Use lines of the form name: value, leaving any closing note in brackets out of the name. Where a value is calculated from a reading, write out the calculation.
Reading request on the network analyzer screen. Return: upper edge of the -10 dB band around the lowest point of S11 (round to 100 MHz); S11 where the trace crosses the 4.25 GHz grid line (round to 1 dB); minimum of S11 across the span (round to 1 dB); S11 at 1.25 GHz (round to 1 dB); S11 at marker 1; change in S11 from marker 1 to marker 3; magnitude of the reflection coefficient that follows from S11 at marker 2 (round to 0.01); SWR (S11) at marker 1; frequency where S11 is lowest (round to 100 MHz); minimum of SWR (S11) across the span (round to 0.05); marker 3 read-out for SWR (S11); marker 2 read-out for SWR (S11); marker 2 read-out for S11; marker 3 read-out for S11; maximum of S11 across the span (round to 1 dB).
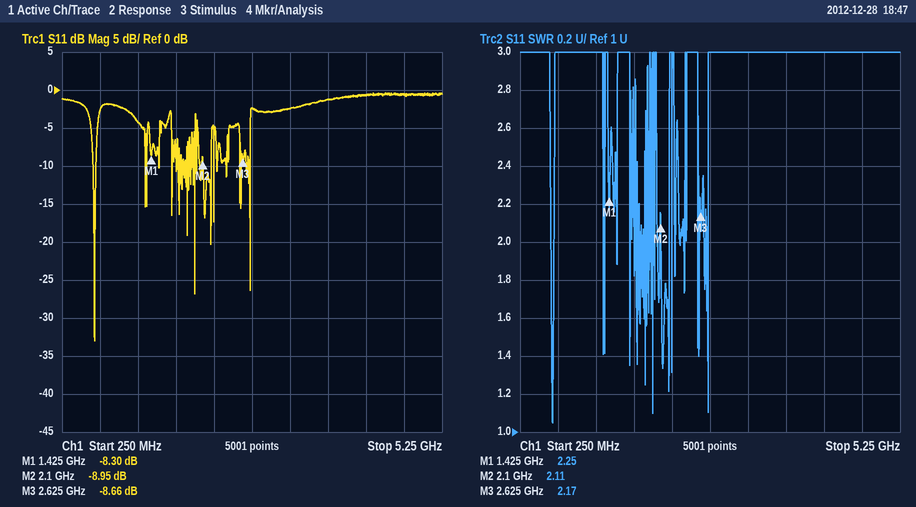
upper edge of the -10 dB band around the lowest point of S11: 700 MHz
S11 where the trace crosses the 4.25 GHz grid line: -1 dB
minimum of S11 across the span: -33 dB
S11 at 1.25 GHz: -4 dB
S11 at marker 1: -8.30 dB
change in S11 from marker 1 to marker 3: -8.66 − (-8.3) = -0.36 dB
magnitude of the reflection coefficient that follows from S11 at marker 2: 10^(-8.95/20) ≈ 0.36
SWR (S11) at marker 1: 2.25
frequency where S11 is lowest: 700 MHz
minimum of SWR (S11) across the span: 1.05
marker 3 read-out for SWR: 2.17
marker 2 read-out for SWR: 2.11
marker 2 read-out for S11: -8.95 dB
marker 3 read-out for S11: -8.66 dB
maximum of S11 across the span: 0 dB
